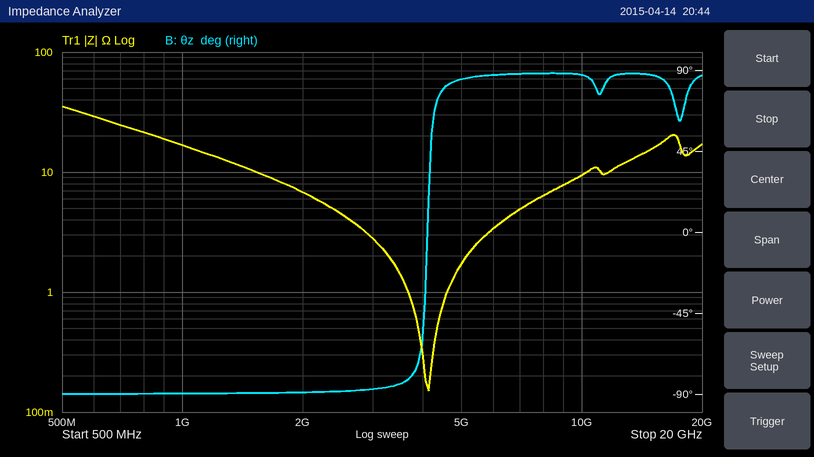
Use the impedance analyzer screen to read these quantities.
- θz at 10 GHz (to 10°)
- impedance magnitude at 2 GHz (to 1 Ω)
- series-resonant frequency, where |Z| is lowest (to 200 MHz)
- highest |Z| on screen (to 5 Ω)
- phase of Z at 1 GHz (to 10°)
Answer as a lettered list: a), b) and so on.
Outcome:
a) 90°
b) 7 Ω
c) 4.2 GHz
d) 35 Ω
e) -90°
